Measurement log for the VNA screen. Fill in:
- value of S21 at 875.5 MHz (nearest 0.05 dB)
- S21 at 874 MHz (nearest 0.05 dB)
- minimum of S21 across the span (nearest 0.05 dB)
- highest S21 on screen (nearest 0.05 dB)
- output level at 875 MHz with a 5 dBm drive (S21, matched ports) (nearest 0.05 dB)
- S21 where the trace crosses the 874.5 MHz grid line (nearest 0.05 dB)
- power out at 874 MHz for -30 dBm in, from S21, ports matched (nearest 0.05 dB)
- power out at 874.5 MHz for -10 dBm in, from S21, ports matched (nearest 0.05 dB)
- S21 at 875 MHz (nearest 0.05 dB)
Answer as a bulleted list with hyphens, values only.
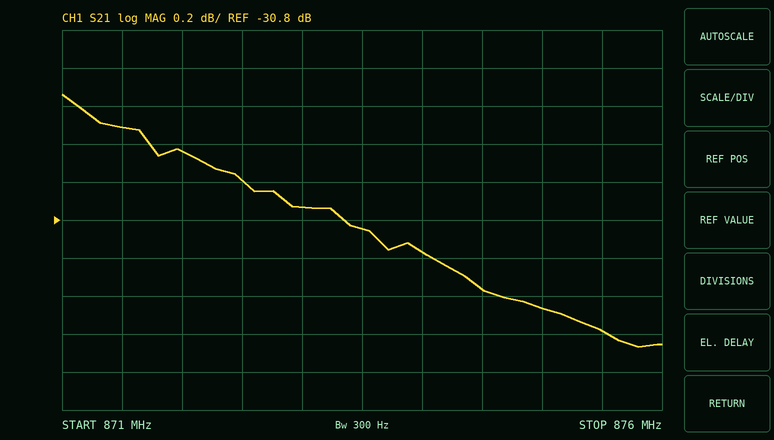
- -31.40 dB
- -30.95 dB
- -31.45 dB
- -30.15 dB
- -26.25 dBm
- -31.15 dB
- -60.95 dBm
- -41.15 dBm
- -31.25 dB
